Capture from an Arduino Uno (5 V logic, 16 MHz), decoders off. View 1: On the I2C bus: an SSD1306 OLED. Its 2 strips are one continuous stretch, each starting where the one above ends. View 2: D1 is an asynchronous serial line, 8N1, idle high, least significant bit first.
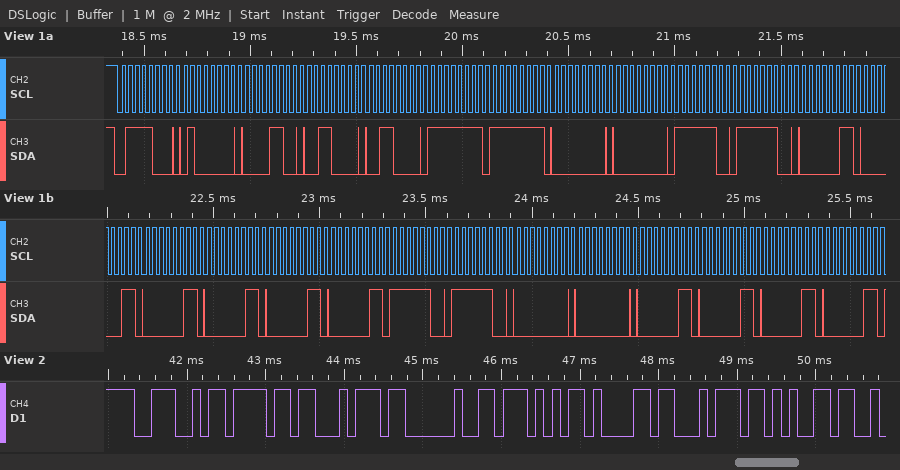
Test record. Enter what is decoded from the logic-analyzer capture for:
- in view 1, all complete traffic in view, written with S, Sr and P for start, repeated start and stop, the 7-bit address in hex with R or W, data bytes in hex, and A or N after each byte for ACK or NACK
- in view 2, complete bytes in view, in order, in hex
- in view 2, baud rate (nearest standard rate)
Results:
S 3CW A 40 A 0C A 30 A 30 A FF A FF A 00 A 00 A FC A FC A 03 A 03 A 03 A 03 A 03 A 03 A FC A FC A 00 A 00 A 03 A 03 A 03 A 03 A
4E 6F 74 20 57 61 74 65
9600 baud
